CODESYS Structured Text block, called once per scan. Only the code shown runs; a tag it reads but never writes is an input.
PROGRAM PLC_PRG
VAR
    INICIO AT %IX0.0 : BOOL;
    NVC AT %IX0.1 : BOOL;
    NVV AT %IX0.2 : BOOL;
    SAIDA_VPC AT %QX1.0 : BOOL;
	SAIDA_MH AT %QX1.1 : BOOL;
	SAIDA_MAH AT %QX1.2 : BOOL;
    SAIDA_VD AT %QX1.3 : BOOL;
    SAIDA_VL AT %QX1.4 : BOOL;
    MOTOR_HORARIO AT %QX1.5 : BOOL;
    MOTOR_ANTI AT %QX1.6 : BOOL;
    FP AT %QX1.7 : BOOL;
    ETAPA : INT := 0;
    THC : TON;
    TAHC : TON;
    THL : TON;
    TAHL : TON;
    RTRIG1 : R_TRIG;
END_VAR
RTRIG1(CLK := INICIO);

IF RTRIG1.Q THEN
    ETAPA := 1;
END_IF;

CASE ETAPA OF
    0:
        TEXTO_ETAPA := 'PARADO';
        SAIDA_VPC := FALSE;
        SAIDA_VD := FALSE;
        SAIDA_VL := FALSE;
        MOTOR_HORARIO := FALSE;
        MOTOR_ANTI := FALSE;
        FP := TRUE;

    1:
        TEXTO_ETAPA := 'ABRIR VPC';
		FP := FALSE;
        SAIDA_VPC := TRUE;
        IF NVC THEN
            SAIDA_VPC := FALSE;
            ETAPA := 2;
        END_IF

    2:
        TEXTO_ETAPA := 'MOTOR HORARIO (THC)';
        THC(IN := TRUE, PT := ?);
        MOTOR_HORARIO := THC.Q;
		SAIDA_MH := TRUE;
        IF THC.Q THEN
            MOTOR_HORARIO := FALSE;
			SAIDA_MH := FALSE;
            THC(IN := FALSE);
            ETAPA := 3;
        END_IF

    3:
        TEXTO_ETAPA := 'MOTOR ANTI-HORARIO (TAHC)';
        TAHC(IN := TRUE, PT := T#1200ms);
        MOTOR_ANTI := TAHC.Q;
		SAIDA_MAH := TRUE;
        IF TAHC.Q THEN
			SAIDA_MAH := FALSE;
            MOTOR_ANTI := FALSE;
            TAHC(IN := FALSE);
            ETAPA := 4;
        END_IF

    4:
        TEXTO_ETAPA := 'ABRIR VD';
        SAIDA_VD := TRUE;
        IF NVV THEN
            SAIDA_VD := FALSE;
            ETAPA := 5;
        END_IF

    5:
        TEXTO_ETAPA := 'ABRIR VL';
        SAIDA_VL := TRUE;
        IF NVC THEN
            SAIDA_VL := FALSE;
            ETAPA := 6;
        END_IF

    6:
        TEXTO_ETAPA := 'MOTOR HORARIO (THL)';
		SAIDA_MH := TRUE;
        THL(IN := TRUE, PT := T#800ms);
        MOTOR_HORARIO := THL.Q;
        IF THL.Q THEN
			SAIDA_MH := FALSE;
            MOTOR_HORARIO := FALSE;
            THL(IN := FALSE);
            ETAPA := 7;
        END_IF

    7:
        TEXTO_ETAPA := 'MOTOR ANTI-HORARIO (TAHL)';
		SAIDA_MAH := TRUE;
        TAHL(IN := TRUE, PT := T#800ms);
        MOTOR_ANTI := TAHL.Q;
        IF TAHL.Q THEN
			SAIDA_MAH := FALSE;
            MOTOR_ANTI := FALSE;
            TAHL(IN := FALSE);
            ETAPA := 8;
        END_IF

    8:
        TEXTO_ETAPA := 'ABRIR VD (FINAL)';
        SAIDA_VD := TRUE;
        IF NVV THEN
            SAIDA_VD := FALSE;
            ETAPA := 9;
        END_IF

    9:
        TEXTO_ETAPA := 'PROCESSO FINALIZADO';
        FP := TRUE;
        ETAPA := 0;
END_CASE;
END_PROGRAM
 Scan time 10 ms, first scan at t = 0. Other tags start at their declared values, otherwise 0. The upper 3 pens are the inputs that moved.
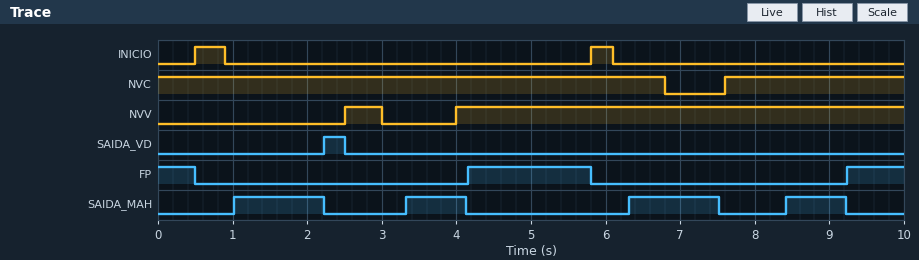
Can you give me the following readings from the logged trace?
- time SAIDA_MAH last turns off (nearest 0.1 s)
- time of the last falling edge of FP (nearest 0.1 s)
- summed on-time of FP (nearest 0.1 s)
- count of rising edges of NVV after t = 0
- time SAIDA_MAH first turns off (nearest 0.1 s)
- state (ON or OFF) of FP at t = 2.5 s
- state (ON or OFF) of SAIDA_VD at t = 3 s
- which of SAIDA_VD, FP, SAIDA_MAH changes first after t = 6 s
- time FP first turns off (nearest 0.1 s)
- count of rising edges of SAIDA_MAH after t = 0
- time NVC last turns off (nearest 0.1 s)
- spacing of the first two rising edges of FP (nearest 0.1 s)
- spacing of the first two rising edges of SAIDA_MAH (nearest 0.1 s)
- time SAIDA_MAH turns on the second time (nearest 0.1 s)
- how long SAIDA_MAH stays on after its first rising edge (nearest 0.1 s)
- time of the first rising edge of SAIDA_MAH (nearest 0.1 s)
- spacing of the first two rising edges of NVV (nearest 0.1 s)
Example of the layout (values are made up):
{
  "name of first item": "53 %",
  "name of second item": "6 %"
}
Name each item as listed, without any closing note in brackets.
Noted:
{
  "time SAIDA_MAH last turns off": "9.2 s",
  "time of the last falling edge of FP": "5.8 s",
  "summed on-time of FP": "2.9 s",
  "count of rising edges of NVV after t = 0": "2",
  "time SAIDA_MAH first turns off": "2.2 s",
  "state (ON or OFF) of FP at t = 2.5 s": "OFF",
  "state (ON or OFF) of SAIDA_VD at t = 3 s": "OFF",
  "which of SAIDA_VD, FP, SAIDA_MAH changes first after t = 6 s": "SAIDA_MAH",
  "time FP first turns off": "0.5 s",
  "count of rising edges of SAIDA_MAH after t = 0": "4",
  "time NVC last turns off": "6.8 s",
  "spacing of the first two rising edges of FP": "5.1 s",
  "spacing of the first two rising edges of SAIDA_MAH": "2.3 s",
  "time SAIDA_MAH turns on the second time": "3.3 s",
  "how long SAIDA_MAH stays on after its first rising edge": "1.2 s",
  "time of the first rising edge of SAIDA_MAH": "1.0 s",
  "spacing of the first two rising edges of NVV": "1.5 s"
}
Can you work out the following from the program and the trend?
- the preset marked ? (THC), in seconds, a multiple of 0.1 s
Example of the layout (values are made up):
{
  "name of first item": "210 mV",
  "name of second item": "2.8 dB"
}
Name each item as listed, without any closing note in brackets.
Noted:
{
  "the preset marked ? (THC), in seconds, a multiple of 0.1 s": "0.5 s"
}
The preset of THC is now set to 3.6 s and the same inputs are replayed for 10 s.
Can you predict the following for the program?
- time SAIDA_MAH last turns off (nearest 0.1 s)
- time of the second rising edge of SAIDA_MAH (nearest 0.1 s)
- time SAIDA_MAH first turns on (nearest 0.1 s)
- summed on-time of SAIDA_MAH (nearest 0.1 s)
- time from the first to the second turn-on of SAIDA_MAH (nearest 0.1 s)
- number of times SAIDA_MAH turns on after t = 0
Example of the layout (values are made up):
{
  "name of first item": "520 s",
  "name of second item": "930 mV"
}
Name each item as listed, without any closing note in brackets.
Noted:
{
  "time SAIDA_MAH last turns off": "5.3 s",
  "time of the second rising edge of SAIDA_MAH": "9.4 s",
  "time SAIDA_MAH first turns on": "4.1 s",
  "summed on-time of SAIDA_MAH": "1.8 s",
  "time from the first to the second turn-on of SAIDA_MAH": "5.3 s",
  "number of times SAIDA_MAH turns on after t = 0": "2"
}
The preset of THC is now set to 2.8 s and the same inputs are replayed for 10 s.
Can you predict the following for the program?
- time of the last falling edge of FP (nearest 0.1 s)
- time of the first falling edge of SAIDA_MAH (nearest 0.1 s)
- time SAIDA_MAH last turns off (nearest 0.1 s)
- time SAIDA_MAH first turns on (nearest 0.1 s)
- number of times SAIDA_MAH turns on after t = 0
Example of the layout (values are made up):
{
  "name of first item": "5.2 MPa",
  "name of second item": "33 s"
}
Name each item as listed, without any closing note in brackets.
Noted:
{
  "time of the last falling edge of FP": "0.5 s",
  "time of the first falling edge of SAIDA_MAH": "4.5 s",
  "time SAIDA_MAH last turns off": "9.8 s",
  "time SAIDA_MAH first turns on": "3.3 s",
  "number of times SAIDA_MAH turns on after t = 0": "2"
}
